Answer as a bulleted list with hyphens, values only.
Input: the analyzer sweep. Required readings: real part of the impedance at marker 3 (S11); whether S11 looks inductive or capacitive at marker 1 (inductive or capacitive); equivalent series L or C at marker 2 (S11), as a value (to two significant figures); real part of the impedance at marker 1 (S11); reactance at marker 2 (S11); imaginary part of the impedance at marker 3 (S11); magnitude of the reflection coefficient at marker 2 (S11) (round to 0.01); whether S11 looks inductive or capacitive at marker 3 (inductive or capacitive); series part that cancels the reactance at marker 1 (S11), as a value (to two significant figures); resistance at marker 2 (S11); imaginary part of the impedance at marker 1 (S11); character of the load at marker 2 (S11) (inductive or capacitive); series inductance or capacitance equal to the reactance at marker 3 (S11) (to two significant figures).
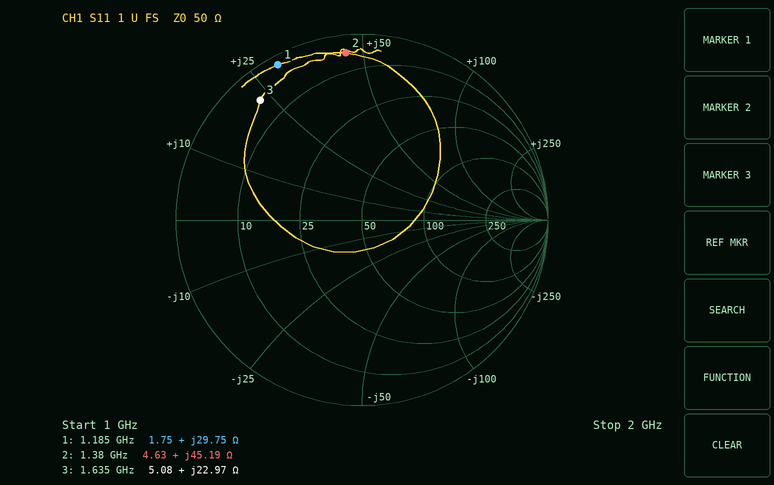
- 5.08 Ω
- inductive
- 5.2 nH
- 1.75 Ω
- +45.19 Ω
- +22.97 Ω
- 0.90
- inductive
- 4.5 pF
- 4.63 Ω
- +29.75 Ω
- inductive
- 2.2 nH
